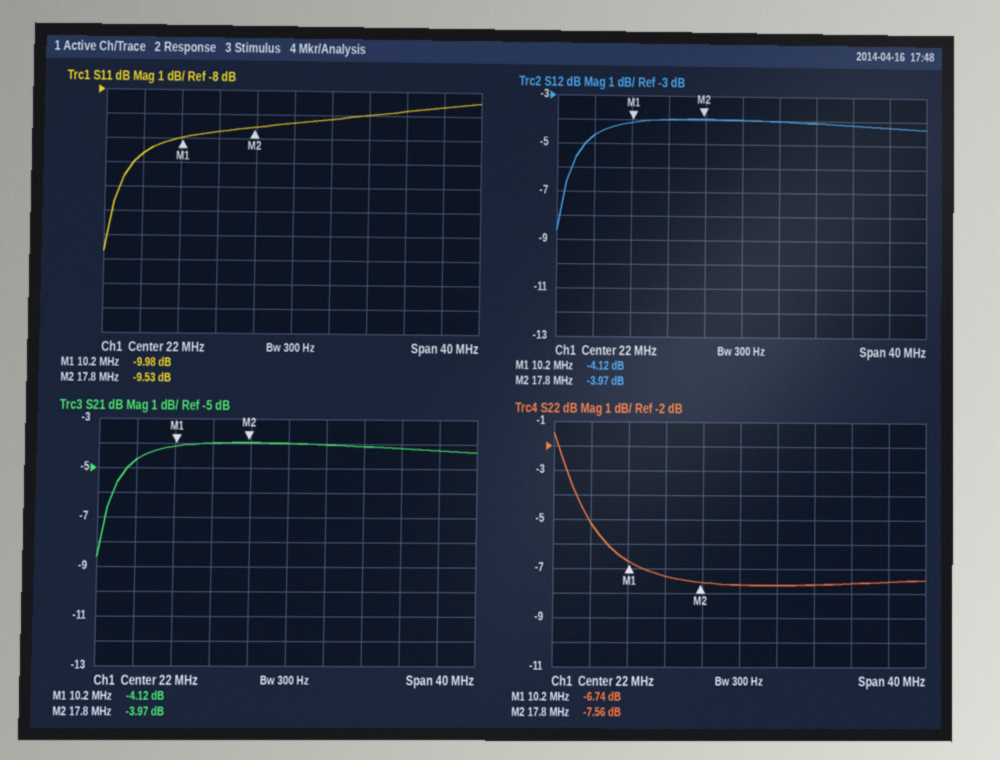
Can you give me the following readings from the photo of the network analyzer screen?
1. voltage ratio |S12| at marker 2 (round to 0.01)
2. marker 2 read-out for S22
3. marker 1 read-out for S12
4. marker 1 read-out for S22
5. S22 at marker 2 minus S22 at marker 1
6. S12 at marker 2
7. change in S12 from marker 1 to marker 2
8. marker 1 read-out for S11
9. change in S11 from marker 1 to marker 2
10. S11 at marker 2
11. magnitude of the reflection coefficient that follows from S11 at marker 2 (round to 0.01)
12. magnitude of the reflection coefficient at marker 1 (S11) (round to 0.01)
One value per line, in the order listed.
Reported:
0.63
-7.56 dB
-4.12 dB
-6.74 dB
-0.82 dB
-3.97 dB
0.15 dB
-9.98 dB
0.45 dB
-9.53 dB
0.33
0.32
